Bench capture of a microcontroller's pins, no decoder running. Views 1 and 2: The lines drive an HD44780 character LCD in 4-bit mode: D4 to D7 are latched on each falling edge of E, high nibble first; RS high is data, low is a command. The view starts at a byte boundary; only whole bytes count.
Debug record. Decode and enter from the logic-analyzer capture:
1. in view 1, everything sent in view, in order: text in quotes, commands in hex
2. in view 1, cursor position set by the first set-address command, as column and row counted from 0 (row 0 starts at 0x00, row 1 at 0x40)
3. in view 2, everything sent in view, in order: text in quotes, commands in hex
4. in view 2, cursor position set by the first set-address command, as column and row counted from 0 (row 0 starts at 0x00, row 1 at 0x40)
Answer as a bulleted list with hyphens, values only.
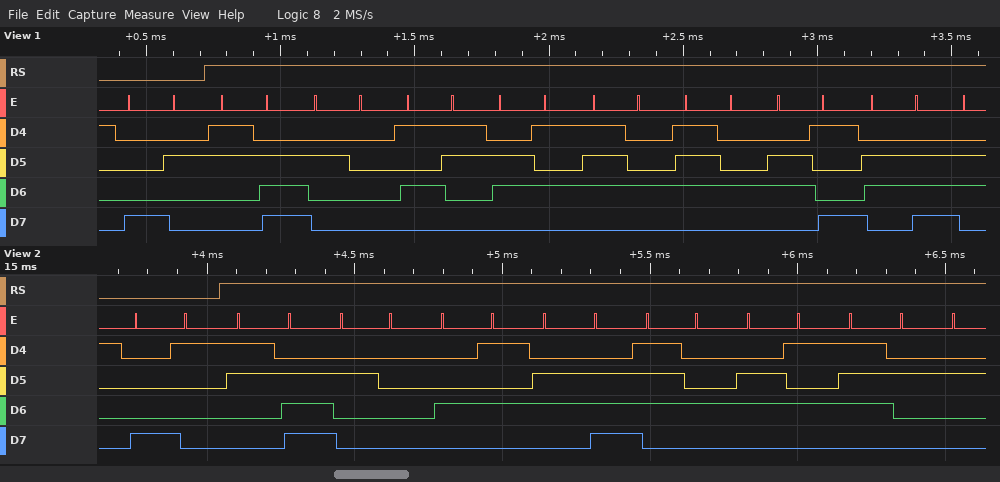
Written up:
- 0x82 "> Settin"
- column 2, row 0
- 0x81 "> Enter"
- column 1, row 0
